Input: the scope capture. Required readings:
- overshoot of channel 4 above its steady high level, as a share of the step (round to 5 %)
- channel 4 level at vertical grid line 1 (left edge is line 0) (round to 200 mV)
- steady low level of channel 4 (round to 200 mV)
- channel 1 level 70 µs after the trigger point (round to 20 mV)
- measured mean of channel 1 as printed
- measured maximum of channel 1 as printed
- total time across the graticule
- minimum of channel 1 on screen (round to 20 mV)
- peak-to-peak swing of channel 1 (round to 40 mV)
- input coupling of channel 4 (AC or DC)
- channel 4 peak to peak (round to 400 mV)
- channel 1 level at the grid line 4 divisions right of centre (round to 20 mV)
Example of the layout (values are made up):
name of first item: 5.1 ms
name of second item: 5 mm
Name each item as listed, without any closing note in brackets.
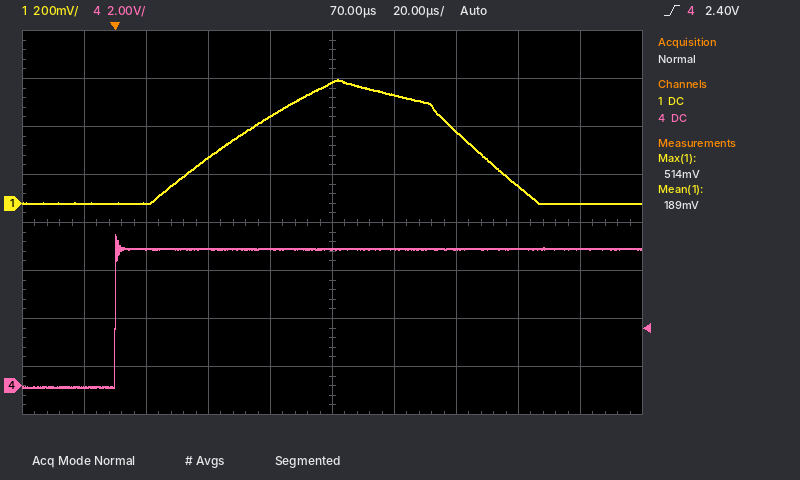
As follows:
overshoot of channel 4 above its steady high level, as a share of the step: 10 %
channel 4 level at vertical grid line 1 (left edge is line 0): 0.0 V
steady low level of channel 4: 0.0 V
channel 1 level 70 µs after the trigger point: 500 mV
measured mean of channel 1 as printed: 189 mV
measured maximum of channel 1 as printed: 514 mV
total time across the graticule: 200 µs
minimum of channel 1 on screen: 0 mV
peak-to-peak swing of channel 1: 520 mV
input coupling of channel 4: DC
channel 4 peak to peak: 6.4 V
channel 1 level at the grid line 4 divisions right of centre: 0 mV
